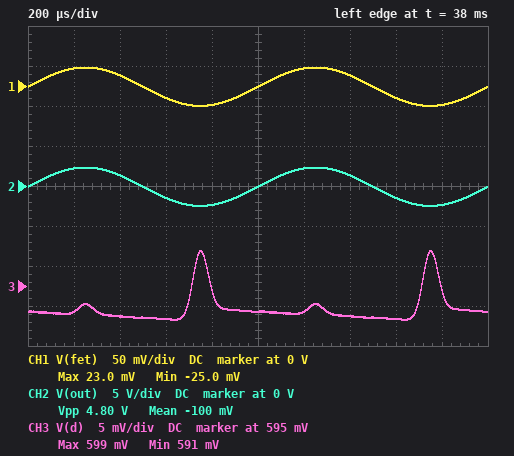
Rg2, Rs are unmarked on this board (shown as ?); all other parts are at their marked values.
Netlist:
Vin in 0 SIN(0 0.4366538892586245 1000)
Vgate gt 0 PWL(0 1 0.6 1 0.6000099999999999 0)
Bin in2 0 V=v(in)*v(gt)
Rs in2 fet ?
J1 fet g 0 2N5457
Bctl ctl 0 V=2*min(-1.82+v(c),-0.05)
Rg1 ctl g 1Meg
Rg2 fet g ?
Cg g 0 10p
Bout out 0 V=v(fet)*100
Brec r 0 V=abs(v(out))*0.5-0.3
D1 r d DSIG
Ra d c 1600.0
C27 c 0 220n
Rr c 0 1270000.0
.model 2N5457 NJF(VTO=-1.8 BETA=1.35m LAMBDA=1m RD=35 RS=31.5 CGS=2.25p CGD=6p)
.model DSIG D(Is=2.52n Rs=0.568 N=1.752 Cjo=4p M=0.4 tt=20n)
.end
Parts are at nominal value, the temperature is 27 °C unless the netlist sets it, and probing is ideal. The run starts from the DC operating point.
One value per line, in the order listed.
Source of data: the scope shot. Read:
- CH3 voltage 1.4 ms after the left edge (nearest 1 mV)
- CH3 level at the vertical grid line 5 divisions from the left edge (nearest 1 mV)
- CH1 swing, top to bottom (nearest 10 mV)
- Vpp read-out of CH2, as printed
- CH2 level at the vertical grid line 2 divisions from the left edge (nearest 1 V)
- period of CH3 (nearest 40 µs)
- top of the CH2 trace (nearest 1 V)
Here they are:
591 mV
592 mV
50 mV
4.80 V
1 V
1.00 ms
2 V
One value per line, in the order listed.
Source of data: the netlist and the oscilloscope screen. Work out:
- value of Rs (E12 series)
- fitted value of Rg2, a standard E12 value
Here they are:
15 kΩ
1.2 MΩ
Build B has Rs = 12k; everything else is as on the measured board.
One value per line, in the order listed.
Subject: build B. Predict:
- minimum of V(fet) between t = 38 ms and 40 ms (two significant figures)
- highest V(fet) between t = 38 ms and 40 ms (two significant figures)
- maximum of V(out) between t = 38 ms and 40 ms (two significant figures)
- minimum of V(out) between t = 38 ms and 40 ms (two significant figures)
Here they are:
-26 mV
25 mV
2.5 V
-2.6 V
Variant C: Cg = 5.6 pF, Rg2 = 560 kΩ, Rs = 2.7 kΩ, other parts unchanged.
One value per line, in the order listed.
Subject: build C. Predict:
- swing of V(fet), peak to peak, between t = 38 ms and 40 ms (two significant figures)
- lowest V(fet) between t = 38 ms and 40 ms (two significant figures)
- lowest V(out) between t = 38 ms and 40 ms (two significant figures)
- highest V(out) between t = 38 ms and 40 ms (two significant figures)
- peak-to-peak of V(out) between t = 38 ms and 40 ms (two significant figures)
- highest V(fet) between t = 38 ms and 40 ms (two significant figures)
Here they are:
88 mV
-44 mV
-4.4 V
4.4 V
8.8 V
44 mV
